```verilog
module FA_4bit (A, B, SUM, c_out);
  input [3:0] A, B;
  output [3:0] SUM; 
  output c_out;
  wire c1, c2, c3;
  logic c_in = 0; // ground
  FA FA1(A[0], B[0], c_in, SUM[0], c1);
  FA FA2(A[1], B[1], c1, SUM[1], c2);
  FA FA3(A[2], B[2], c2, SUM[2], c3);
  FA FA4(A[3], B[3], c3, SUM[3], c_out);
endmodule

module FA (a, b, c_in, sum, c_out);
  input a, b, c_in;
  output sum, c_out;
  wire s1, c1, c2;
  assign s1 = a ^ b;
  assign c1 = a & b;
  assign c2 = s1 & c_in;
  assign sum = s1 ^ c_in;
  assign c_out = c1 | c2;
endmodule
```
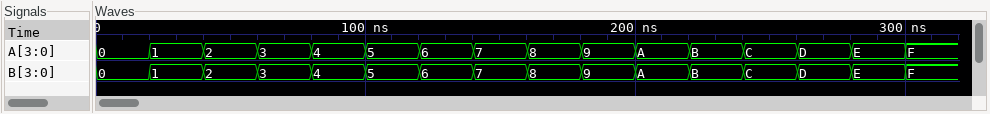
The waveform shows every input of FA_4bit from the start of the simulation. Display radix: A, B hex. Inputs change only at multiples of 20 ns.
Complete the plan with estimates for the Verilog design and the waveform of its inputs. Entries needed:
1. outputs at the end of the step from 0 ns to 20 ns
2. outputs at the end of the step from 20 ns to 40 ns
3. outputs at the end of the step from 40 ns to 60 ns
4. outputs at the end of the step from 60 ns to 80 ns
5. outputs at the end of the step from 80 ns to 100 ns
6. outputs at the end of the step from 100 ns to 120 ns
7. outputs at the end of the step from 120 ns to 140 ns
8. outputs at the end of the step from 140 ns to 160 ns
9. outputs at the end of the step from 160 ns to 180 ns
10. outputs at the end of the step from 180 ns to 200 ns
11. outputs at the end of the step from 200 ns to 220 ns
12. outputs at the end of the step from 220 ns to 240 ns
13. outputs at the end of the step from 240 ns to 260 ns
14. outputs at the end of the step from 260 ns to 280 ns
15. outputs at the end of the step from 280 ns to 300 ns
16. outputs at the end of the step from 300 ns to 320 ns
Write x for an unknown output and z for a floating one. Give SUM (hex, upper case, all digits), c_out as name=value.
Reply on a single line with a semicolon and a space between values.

SUM=0, c_out=0; SUM=2, c_out=0; SUM=4, c_out=0; SUM=6, c_out=0; SUM=8, c_out=0; SUM=A, c_out=0; SUM=C, c_out=0; SUM=E, c_out=0; SUM=0, c_out=1; SUM=2, c_out=1; SUM=4, c_out=1; SUM=6, c_out=1; SUM=8, c_out=1; SUM=A, c_out=1; SUM=C, c_out=1; SUM=E, c_out=1
